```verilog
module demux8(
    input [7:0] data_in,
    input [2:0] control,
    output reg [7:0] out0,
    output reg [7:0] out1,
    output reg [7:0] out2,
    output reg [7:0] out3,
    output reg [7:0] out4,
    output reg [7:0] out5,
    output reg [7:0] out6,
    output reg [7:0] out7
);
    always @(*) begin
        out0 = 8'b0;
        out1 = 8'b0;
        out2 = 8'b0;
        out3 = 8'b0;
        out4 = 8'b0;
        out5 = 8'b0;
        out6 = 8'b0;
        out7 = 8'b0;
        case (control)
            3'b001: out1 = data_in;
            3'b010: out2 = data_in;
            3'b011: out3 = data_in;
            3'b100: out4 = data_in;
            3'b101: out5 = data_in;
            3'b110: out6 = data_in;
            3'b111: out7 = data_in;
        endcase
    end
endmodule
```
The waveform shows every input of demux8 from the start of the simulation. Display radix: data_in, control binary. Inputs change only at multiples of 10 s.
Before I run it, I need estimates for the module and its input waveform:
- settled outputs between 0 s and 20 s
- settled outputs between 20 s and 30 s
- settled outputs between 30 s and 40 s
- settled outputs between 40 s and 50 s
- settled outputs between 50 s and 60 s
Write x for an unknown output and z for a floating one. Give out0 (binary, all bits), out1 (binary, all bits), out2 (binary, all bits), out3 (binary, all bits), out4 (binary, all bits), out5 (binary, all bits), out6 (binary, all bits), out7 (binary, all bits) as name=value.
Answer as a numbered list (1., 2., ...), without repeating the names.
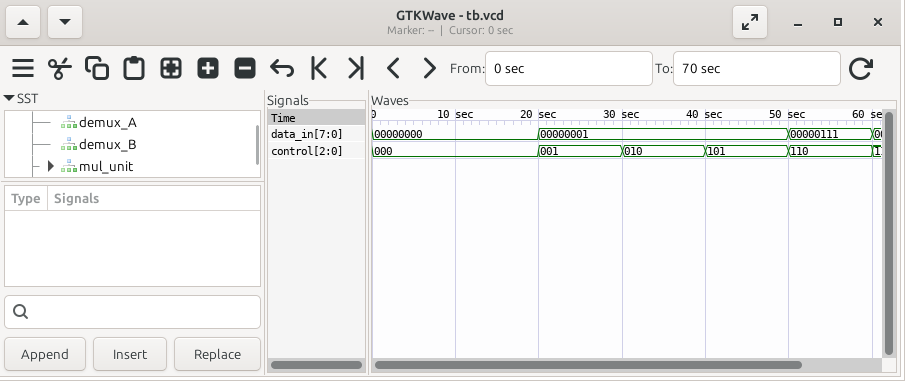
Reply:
1. out0=00000000, out1=00000000, out2=00000000, out3=00000000, out4=00000000, out5=00000000, out6=00000000, out7=00000000
2. out0=00000000, out1=00000001, out2=00000000, out3=00000000, out4=00000000, out5=00000000, out6=00000000, out7=00000000
3. out0=00000000, out1=00000000, out2=00000001, out3=00000000, out4=00000000, out5=00000000, out6=00000000, out7=00000000
4. out0=00000000, out1=00000000, out2=00000000, out3=00000000, out4=00000000, out5=00000001, out6=00000000, out7=00000000
5. out0=00000000, out1=00000000, out2=00000000, out3=00000000, out4=00000000, out5=00000000, out6=00000111, out7=00000000
